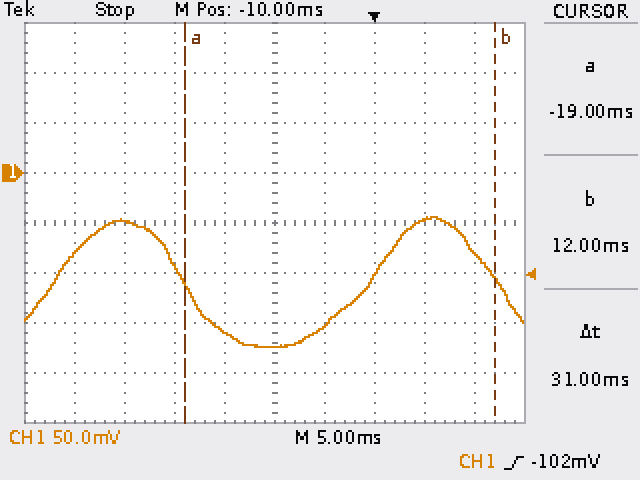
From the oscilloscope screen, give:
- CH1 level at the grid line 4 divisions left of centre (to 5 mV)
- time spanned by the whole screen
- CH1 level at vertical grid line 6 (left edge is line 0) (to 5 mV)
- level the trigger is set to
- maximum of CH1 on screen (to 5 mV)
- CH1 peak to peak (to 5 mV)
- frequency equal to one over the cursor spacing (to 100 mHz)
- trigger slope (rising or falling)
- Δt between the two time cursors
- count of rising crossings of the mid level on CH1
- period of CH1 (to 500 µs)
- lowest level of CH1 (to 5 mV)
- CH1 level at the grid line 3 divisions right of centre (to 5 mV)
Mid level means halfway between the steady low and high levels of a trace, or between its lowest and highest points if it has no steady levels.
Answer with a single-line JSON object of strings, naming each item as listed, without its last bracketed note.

{"CH1 level at the grid line 4 divisions left of centre": "-80 mV", "time spanned by the whole screen": "50 ms", "CH1 level at vertical grid line 6 (left edge is line 0)": "-155 mV", "level the trigger is set to": "-102 mV", "maximum of CH1 on screen": "-45 mV", "CH1 peak to peak": "130 mV", "frequency equal to one over the cursor spacing": "32.3 Hz", "trigger slope": "rising", "Δt between the two time cursors": "31 ms", "count of rising crossings of the mid level on CH1": "2", "period of CH1": "31.5 ms", "lowest level of CH1": "-175 mV", "CH1 level at the grid line 3 divisions right of centre": "-45 mV"}
